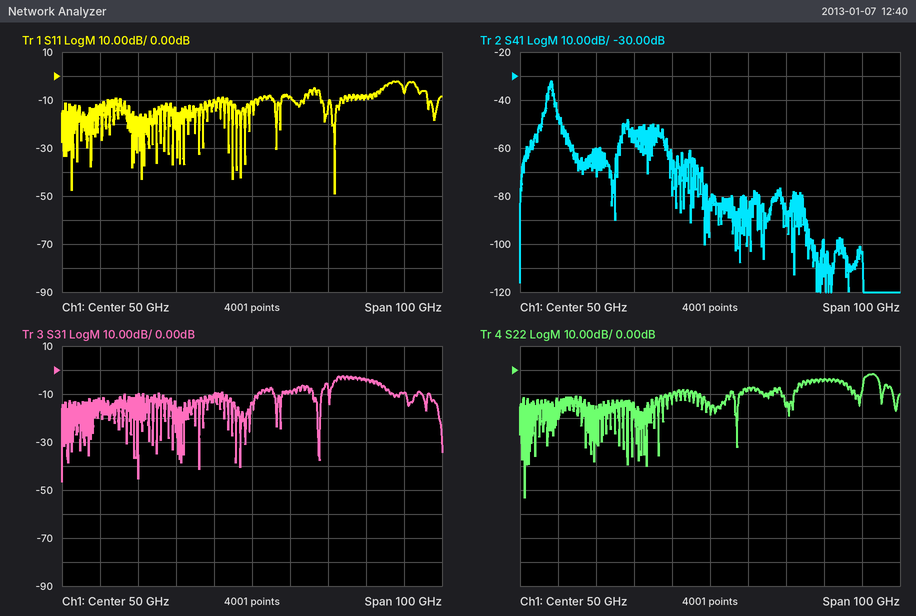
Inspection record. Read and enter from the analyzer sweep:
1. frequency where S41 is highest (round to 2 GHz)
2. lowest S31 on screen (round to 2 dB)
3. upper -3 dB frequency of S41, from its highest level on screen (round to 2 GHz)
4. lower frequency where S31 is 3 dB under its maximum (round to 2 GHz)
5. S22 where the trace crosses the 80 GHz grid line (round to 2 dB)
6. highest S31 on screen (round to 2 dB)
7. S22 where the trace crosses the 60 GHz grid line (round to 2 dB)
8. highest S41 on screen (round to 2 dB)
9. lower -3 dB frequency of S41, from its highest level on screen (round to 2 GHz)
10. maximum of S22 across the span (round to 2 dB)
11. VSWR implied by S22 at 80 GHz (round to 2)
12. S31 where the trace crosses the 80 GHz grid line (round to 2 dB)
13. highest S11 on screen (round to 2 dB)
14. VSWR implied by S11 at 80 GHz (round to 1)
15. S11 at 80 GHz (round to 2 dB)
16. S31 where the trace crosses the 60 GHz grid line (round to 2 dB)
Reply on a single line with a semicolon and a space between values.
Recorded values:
8 GHz; -46 dB; 8 GHz; 72 GHz; -4 dB; -2 dB; -8 dB; -32 dB; 8 GHz; -2 dB; 4; -4 dB; -2 dB; 2; -8 dB; -8 dB
